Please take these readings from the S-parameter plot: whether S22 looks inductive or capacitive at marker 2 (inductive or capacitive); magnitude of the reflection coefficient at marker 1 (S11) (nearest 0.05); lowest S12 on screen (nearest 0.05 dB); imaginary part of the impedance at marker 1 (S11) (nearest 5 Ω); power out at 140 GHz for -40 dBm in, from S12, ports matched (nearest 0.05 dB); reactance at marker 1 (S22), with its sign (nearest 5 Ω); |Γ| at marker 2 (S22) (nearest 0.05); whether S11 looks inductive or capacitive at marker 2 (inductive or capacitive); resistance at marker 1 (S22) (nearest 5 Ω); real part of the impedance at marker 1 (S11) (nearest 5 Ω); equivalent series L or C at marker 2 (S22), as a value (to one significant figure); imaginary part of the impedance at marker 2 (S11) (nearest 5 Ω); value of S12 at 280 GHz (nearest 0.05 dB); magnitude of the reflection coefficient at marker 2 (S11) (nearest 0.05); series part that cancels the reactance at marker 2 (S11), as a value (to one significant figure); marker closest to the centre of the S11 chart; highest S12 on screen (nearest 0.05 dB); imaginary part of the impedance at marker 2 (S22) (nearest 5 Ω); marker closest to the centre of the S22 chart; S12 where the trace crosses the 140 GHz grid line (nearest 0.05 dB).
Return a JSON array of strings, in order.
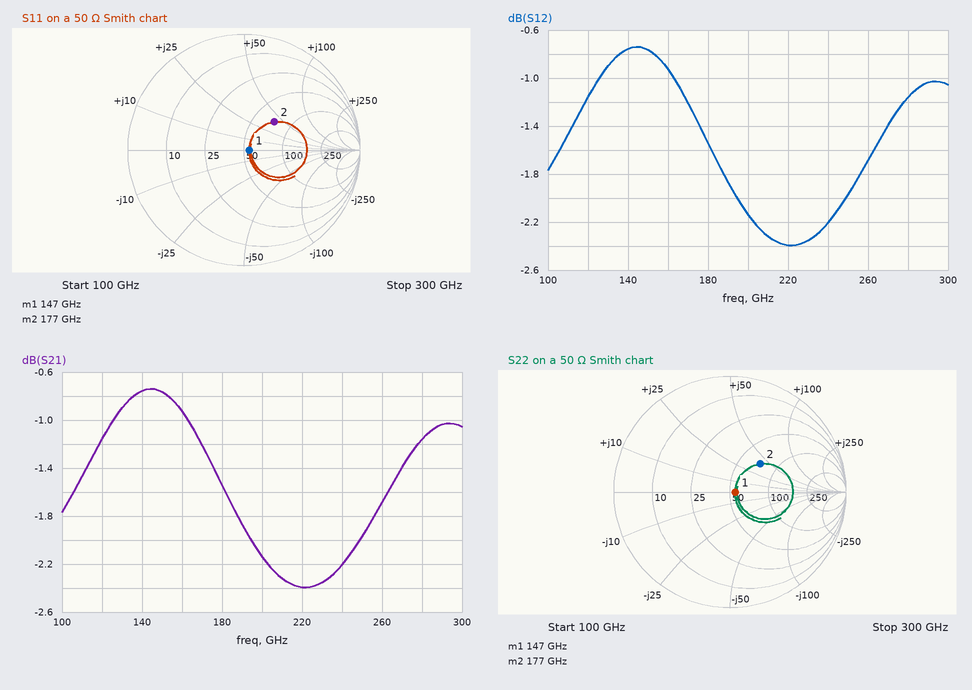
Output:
["inductive", "0.05", "-2.40 dB", "0 Ω", "-40.75 dBm", "0 Ω", "0.35", "inductive", "55 Ω", "55 Ω", "40 pH", "+40 Ω", "-1.15 dB", "0.35", "20 fF", "marker 1", "-0.75 dB", "+40 Ω", "marker 1", "-0.75 dB"]
